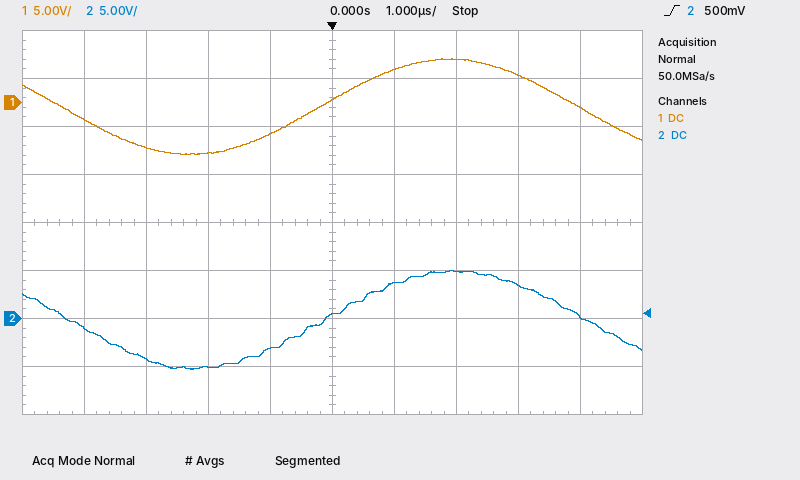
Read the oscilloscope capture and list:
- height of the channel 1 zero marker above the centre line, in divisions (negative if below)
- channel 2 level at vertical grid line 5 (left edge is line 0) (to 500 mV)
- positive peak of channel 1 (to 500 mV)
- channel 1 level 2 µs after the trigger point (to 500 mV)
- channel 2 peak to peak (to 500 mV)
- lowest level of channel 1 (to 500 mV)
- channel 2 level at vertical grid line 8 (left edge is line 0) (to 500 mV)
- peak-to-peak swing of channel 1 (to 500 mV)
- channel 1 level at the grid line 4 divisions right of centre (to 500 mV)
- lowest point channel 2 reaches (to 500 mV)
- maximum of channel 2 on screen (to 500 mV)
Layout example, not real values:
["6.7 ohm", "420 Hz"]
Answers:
["+2.5 div", "500 mV", "4.5 V", "4.5 V", "10.5 V", "-5.5 V", "3.5 V", "10.0 V", "-500 mV", "-5.5 V", "5.0 V"]
